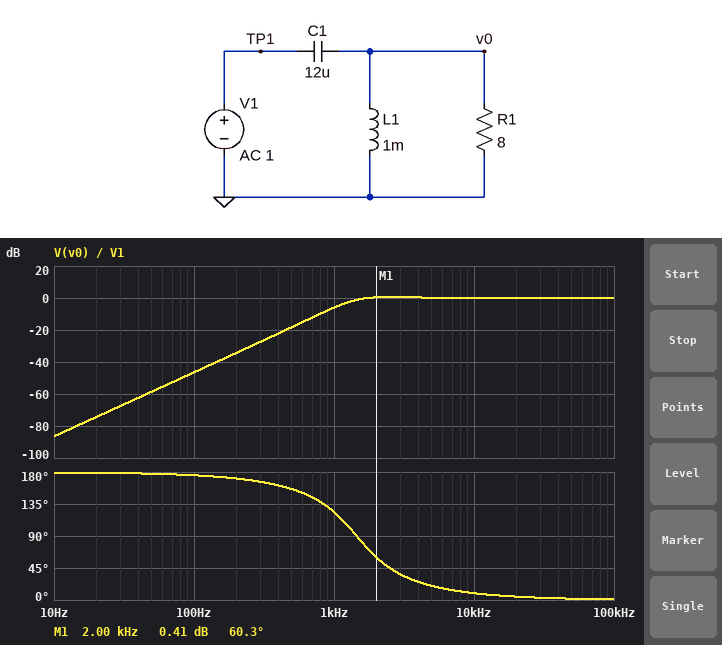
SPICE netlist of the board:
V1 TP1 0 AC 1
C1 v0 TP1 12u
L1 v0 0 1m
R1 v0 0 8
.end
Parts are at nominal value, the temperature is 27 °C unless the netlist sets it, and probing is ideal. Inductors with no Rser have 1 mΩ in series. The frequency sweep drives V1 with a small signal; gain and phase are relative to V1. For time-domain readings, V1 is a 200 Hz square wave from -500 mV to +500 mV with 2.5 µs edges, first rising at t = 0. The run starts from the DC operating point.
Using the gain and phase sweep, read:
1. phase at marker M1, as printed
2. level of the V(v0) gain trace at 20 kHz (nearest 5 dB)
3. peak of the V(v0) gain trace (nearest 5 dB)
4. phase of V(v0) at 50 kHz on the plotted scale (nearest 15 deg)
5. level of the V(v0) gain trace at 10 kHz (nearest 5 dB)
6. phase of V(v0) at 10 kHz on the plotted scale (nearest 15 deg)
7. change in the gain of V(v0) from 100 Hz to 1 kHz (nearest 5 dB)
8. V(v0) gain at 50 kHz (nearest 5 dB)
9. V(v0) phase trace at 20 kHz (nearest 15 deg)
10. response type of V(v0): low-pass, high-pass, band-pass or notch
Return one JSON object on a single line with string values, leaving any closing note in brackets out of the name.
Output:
{"phase at marker M1, as printed": "60.3 deg", "level of the V(v0) gain trace at 20 kHz": "0 dB", "peak of the V(v0) gain trace": "0 dB", "phase of V(v0) at 50 kHz on the plotted scale": "0 deg", "level of the V(v0) gain trace at 10 kHz": "0 dB", "phase of V(v0) at 10 kHz on the plotted scale": "15 deg", "change in the gain of V(v0) from 100 Hz to 1 kHz": "40 dB", "V(v0) gain at 50 kHz": "0 dB", "V(v0) phase trace at 20 kHz": "0 deg", "response type of V(v0): low-pass, high-pass, band-pass or notch": "high-pass"}
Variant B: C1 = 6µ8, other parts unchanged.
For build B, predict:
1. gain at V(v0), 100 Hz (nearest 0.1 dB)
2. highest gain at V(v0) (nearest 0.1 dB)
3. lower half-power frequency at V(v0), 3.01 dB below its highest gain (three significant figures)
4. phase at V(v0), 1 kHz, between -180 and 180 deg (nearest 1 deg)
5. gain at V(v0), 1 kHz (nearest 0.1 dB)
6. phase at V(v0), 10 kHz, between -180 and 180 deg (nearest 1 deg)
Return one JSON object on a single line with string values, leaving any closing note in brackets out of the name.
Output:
{"gain at V(v0), 100 Hz": "-51.4 dB", "highest gain at V(v0)": "0 dB", "lower half-power frequency at V(v0), 3.01 dB below its highest gain": "2.08 kHz", "phase at V(v0), 1 kHz, between -180 and 180 deg": "133 deg", "gain at V(v0), 1 kHz": "-12.0 dB", "phase at V(v0), 10 kHz, between -180 and 180 deg": "17 deg"}
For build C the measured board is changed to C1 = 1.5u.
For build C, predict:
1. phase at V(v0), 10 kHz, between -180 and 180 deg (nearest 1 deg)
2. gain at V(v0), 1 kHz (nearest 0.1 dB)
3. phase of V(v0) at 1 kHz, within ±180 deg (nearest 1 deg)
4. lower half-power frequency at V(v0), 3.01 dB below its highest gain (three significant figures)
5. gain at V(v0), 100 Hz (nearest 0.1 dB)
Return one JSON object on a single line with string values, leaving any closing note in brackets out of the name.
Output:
{"phase at V(v0), 10 kHz, between -180 and 180 deg": "58 deg", "gain at V(v0), 1 kHz": "-26.3 dB", "phase of V(v0) at 1 kHz, within ±180 deg": "140 deg", "lower half-power frequency at V(v0), 3.01 dB below its highest gain": "12.0 kHz", "gain at V(v0), 100 Hz": "-64.6 dB"}
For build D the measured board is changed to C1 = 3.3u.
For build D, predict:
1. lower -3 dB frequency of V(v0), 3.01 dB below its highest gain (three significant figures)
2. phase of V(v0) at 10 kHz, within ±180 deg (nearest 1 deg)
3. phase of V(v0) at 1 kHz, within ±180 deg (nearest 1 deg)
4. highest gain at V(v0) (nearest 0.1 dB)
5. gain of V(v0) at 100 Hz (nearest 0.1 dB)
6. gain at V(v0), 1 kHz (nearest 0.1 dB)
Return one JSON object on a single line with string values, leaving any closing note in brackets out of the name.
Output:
{"lower -3 dB frequency of V(v0), 3.01 dB below its highest gain": "4.85 kHz", "phase of V(v0) at 10 kHz, within ±180 deg": "33 deg", "phase of V(v0) at 1 kHz, within ±180 deg": "138 deg", "highest gain at V(v0)": "0 dB", "gain of V(v0) at 100 Hz": "-57.7 dB", "gain at V(v0), 1 kHz": "-19.1 dB"}
